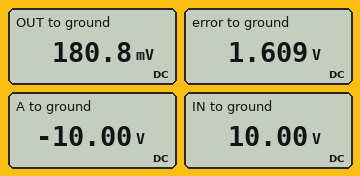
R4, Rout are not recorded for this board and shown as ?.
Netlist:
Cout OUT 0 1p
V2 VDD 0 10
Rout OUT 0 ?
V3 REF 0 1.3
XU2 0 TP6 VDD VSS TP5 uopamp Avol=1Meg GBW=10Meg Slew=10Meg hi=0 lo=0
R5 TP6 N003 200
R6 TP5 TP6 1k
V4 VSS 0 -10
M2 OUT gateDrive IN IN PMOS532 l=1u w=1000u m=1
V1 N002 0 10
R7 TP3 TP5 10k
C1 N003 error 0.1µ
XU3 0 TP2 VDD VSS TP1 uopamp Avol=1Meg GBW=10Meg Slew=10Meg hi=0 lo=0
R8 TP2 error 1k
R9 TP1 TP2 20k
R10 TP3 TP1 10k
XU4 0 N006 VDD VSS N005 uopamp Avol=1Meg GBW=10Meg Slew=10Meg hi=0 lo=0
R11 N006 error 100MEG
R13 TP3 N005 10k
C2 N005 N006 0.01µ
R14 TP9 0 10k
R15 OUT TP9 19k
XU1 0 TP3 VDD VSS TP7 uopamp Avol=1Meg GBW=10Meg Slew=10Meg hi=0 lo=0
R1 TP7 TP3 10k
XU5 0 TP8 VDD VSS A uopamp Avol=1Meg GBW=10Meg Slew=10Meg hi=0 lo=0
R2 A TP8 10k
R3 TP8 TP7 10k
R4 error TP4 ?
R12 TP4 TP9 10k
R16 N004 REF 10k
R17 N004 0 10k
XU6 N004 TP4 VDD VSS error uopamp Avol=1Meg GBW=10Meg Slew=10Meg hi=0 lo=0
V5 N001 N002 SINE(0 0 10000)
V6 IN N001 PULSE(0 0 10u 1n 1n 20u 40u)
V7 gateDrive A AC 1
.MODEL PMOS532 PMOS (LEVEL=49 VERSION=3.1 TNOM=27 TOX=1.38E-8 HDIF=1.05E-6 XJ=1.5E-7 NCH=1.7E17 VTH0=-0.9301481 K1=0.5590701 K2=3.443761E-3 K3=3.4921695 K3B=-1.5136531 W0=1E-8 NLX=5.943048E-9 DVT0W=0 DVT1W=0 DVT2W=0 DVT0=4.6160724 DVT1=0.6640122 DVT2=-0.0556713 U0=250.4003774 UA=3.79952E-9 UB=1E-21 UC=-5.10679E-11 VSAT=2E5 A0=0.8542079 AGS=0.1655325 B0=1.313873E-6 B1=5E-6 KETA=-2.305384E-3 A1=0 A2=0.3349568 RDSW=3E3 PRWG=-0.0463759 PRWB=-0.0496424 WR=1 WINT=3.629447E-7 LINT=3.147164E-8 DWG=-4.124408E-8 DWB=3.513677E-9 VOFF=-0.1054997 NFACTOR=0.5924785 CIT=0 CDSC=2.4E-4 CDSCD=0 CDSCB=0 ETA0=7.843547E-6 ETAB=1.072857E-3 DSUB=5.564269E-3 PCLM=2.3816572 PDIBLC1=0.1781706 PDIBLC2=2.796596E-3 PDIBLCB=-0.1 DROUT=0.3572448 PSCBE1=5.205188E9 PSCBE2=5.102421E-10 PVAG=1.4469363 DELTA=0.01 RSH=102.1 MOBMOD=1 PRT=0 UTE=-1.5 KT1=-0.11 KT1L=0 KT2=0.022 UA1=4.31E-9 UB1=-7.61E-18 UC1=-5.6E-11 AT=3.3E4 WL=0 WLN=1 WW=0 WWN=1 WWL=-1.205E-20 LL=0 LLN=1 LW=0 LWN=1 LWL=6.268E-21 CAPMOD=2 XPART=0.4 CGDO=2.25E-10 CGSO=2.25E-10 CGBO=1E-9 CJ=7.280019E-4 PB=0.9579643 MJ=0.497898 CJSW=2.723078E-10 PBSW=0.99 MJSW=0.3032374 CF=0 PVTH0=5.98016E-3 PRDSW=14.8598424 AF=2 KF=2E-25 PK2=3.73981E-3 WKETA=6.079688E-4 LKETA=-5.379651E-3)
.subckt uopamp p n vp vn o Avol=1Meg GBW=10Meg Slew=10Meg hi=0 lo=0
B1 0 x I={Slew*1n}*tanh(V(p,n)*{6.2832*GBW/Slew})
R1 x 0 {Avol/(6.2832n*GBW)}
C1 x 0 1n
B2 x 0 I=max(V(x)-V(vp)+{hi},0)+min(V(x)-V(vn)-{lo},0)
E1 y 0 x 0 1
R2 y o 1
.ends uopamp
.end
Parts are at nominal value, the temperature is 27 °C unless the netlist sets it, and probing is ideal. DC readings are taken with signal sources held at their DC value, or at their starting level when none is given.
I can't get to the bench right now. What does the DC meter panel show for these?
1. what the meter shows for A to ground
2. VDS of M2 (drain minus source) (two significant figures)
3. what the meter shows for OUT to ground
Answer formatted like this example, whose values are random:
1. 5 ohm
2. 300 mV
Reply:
1. -10.00 V
2. -9.8 V
3. 180.8 mV
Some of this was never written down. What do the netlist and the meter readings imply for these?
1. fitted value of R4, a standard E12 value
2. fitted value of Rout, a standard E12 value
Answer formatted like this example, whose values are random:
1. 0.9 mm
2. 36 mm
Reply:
1. 27 kΩ
2. 3.9 Ω
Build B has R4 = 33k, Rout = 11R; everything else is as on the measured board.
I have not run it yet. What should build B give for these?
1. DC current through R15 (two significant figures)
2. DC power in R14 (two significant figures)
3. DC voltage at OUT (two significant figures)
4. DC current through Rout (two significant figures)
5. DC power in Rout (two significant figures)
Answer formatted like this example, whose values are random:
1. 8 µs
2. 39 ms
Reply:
1. 7.0 µA
2. 13 µW
3. 490 mV
4. 45 mA
5. 22 mW
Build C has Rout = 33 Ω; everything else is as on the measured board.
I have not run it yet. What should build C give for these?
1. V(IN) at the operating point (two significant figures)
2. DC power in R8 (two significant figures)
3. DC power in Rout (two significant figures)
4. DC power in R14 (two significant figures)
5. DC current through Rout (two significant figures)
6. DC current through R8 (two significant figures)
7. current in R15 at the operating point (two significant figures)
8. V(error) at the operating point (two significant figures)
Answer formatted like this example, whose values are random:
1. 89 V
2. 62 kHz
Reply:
1. 10 V
2. 270 µW
3. 55 mW
4. 29 µW
5. 41 mA
6. 520 µA
7. 43 µA
8. 950 mV
